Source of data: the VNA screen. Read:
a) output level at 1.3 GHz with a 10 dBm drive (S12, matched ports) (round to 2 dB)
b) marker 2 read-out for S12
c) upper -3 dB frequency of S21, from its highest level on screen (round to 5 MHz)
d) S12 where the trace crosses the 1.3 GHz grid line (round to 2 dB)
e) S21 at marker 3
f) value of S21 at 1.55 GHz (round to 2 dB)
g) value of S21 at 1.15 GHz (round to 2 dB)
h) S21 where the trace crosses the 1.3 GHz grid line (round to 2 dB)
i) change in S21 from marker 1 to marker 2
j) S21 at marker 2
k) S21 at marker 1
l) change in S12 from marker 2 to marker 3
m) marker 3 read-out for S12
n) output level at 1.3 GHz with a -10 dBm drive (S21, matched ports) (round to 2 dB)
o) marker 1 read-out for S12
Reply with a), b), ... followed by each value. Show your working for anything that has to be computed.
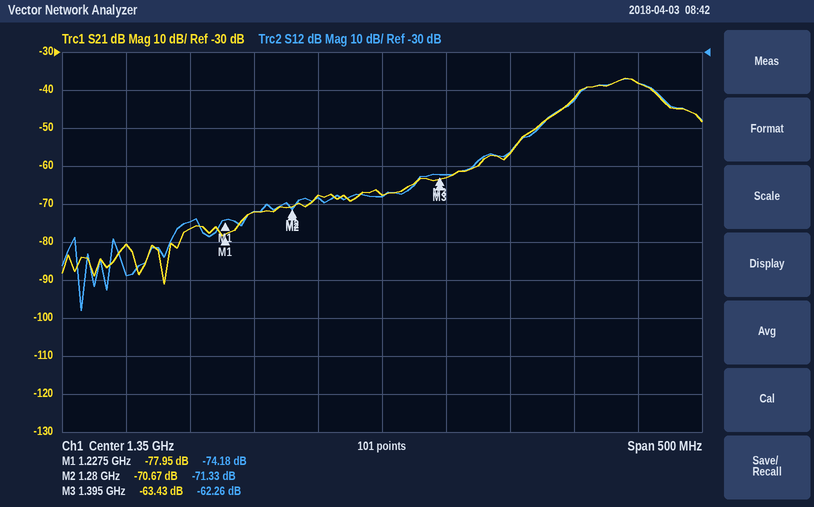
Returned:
a) 10 dBm + (-68 dB) = -58 dBm
b) -71.33 dB
c) 1.560 GHz
d) -68 dB
e) -63.43 dB
f) -38 dB
g) -80 dB
h) -68 dB
i) -70.67 − (-77.95) = 7.28 dB
j) -70.67 dB
k) -77.95 dB
l) -62.26 − (-71.33) = 9.07 dB
m) -62.26 dB
n) -10 dBm + (-68 dB) = -78 dBm
o) -74.18 dB
